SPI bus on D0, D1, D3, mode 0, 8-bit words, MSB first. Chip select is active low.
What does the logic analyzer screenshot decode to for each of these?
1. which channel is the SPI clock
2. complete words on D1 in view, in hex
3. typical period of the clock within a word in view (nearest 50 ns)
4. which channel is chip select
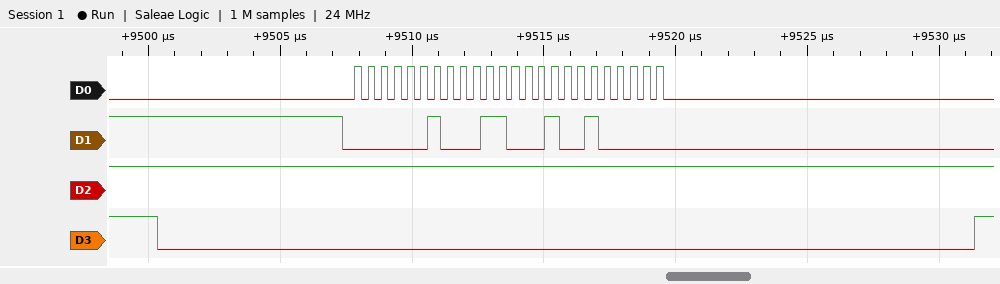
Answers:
D0
02, 31, 20
500 ns
D3
